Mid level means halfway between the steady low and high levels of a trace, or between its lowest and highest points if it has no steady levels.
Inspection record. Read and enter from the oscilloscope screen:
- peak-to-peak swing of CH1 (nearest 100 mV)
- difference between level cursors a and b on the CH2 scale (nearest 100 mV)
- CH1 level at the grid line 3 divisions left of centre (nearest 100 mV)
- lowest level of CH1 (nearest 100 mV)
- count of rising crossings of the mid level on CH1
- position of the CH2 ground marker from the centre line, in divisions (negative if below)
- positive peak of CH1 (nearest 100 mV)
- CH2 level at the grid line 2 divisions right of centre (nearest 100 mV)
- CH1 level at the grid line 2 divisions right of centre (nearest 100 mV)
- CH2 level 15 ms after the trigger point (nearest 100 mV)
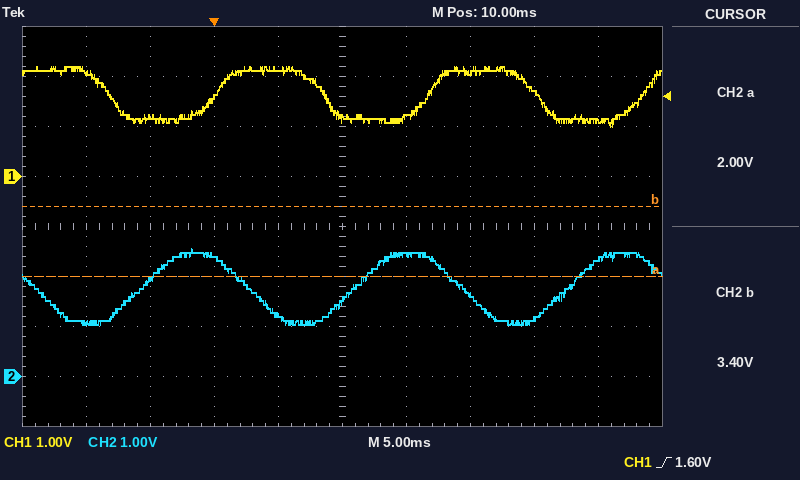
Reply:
1.2 V
1.4 V
1.2 V
1.0 V
3
-3.0 div
2.2 V
1.6 V
2.1 V
2.4 V
